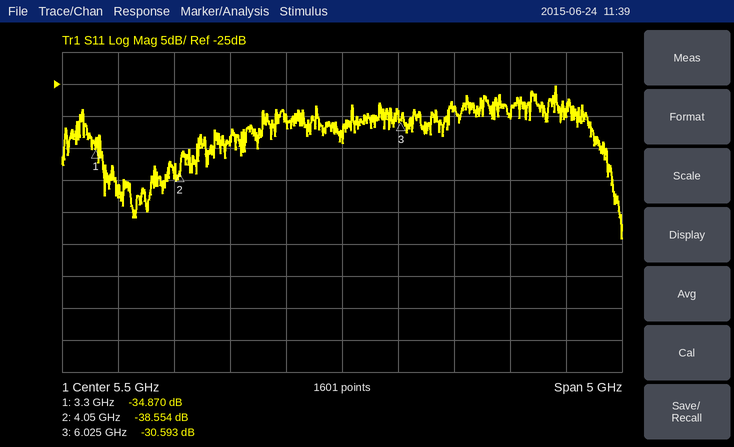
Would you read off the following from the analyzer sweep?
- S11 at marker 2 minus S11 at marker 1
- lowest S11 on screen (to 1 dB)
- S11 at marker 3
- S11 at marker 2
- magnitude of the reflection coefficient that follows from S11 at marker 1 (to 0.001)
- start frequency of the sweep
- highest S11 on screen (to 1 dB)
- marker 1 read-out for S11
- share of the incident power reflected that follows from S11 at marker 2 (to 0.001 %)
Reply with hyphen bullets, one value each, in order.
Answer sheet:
- -3.684 dB
- -49 dB
- -30.593 dB
- -38.554 dB
- 0.018
- 3 GHz
- -25 dB
- -34.870 dB
- 0.014 %
